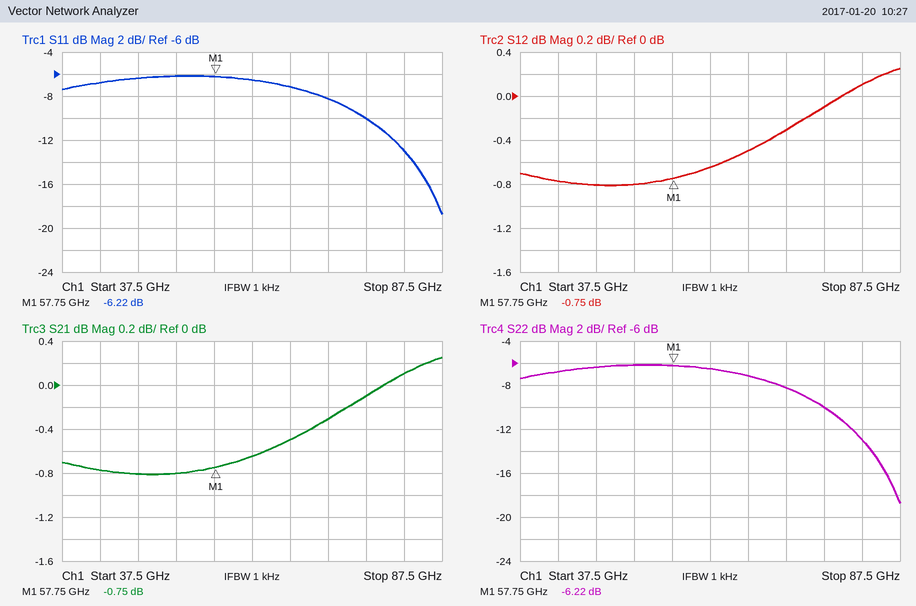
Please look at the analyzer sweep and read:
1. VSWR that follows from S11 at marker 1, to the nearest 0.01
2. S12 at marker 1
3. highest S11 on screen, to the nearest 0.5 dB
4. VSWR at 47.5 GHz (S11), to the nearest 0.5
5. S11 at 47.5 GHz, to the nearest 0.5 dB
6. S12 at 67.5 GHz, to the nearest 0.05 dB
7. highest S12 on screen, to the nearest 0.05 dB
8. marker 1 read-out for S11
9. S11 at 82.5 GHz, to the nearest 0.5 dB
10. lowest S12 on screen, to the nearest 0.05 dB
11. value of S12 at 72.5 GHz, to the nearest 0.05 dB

2.91
-0.75 dB
-6.0 dB
3.0
-6.5 dB
-0.50 dB
0.25 dB
-6.22 dB
-13.0 dB
-0.80 dB
-0.30 dB
